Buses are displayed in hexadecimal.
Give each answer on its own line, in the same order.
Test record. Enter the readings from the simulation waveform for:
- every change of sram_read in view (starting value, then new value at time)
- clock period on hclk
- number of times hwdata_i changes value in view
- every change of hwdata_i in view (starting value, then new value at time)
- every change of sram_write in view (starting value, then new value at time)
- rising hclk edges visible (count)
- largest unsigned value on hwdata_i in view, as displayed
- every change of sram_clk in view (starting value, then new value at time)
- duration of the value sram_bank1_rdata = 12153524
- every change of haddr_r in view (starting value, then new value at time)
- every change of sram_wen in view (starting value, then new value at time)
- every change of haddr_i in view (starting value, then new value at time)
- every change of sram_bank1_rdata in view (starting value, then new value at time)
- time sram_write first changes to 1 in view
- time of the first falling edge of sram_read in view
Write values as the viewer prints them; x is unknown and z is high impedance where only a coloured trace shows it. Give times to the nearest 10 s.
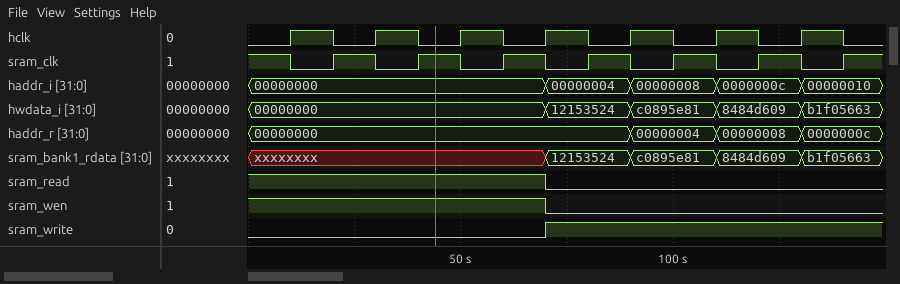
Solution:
1, 0 at 70 s
20 s
4
00000000, 12153524 at 70 s, c0895e81 at 90 s, 8484d609 at 110 s, b1f05663 at 130 s
0, 1 at 70 s
7
c0895e81
1, 0 at 10 s, 1 at 20 s, 0 at 30 s, 1 at 40 s, 0 at 50 s, 1 at 60 s, 0 at 70 s, 1 at 80 s, 0 at 90 s, 1 at 100 s, 0 at 110 s, 1 at 120 s, 0 at 130 s, 1 at 140 s
20 s
00000000, 00000004 at 90 s, 00000008 at 110 s, 0000000c at 130 s
1, 0 at 70 s
00000000, 00000004 at 70 s, 00000008 at 90 s, 0000000c at 110 s, 00000010 at 130 s
xxxxxxxx, 12153524 at 70 s, c0895e81 at 90 s, 8484d609 at 110 s, b1f05663 at 130 s
70 s
70 s
